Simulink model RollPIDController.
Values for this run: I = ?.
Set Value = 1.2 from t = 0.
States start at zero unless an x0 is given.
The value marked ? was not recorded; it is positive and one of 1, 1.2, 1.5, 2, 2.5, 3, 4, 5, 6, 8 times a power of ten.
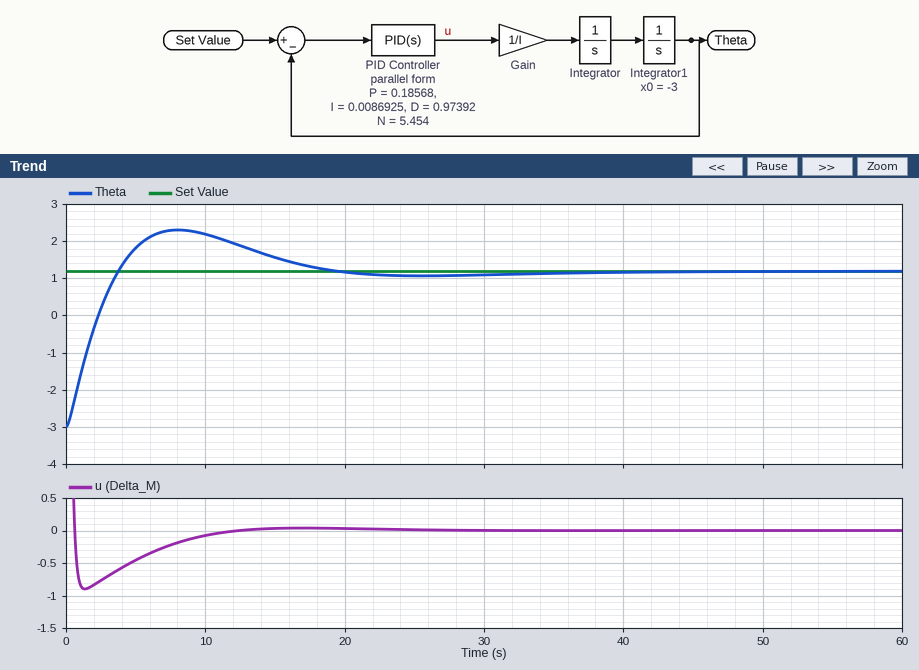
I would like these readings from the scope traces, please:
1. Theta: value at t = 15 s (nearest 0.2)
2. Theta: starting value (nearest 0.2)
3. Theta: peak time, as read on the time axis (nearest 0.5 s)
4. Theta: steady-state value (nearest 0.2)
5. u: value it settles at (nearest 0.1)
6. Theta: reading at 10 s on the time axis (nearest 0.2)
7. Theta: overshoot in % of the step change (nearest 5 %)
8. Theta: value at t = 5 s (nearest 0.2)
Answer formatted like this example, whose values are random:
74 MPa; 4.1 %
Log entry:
1.6; -3.0; 8.0 s; 1.2; 0.0; 2.2; 25 %; 1.8
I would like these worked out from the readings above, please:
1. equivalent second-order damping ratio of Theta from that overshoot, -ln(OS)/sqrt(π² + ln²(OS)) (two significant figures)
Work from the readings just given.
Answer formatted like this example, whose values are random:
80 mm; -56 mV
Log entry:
0.40
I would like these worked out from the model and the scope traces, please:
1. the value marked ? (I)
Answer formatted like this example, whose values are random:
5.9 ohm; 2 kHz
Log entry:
2.5
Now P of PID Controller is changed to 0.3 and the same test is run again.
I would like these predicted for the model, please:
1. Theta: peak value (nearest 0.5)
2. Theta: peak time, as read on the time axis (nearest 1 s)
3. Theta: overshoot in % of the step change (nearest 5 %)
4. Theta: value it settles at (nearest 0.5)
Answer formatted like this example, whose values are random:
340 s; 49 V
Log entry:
2.5; 7 s; 30 %; 1.0
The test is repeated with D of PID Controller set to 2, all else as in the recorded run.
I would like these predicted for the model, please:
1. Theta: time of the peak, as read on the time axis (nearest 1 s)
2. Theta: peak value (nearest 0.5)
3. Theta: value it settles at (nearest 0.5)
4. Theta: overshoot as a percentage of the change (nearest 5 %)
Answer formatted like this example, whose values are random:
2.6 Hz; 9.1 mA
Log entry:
6 s; 1.5; 1.0; 10 %
